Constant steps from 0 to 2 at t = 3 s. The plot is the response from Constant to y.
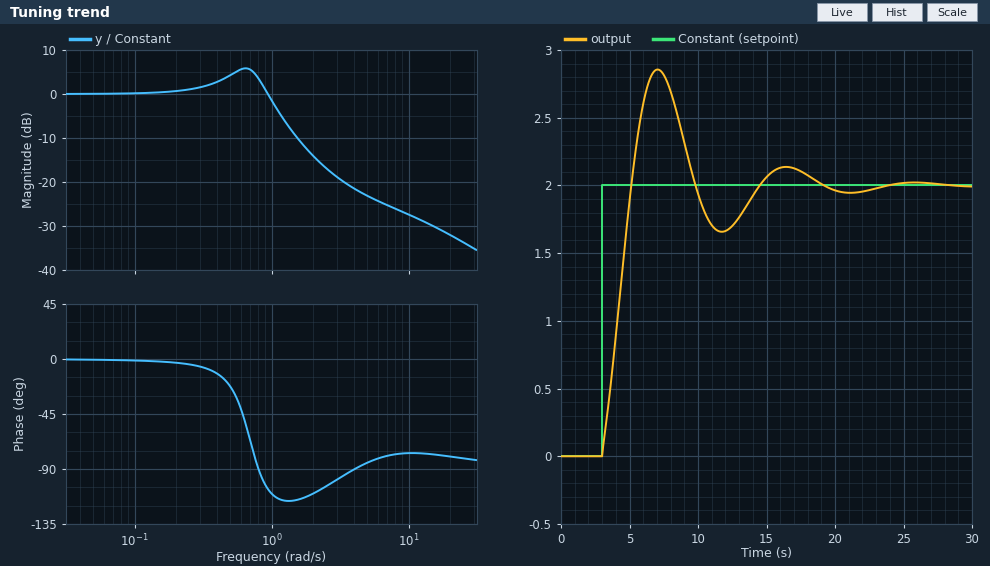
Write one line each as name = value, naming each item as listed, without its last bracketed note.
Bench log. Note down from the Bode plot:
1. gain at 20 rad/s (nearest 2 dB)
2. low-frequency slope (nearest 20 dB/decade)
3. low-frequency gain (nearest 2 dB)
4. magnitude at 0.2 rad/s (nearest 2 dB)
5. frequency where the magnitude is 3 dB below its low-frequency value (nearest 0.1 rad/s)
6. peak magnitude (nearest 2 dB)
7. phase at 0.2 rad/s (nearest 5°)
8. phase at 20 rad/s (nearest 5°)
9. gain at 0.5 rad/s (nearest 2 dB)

gain at 20 rad/s = -32 dB
low-frequency slope = 0 dB/decade
low-frequency gain = 0 dB
magnitude at 0.2 rad/s = 0 dB
frequency where the magnitude is 3 dB below its low-frequency value = 1.1 rad/s
peak magnitude = 6 dB
phase at 0.2 rad/s = -5°
phase at 20 rad/s = -80°
gain at 0.5 rad/s = 4 dB
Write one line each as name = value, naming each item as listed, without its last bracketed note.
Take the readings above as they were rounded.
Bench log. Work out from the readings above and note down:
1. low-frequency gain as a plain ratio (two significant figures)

low-frequency gain as a plain ratio = 1.0
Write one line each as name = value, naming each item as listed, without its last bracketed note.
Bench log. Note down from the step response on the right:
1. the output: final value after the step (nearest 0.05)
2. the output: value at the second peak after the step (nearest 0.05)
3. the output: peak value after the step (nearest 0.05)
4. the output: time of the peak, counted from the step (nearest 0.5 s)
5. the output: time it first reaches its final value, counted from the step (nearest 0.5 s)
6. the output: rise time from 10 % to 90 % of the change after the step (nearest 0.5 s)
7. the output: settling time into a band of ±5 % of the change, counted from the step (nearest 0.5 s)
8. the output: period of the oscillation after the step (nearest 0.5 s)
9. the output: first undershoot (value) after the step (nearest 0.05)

the output: final value after the step = 2.00
the output: value at the second peak after the step = 2.15
the output: peak value after the step = 2.85
the output: time of the peak, counted from the step = 4.0 s
the output: time it first reaches its final value, counted from the step = 2.0 s
the output: rise time from 10 % to 90 % of the change after the step = 1.5 s
the output: settling time into a band of ±5 % of the change, counted from the step = 14.5 s
the output: period of the oscillation after the step = 9.5 s
the output: first undershoot (value) after the step = 1.65
